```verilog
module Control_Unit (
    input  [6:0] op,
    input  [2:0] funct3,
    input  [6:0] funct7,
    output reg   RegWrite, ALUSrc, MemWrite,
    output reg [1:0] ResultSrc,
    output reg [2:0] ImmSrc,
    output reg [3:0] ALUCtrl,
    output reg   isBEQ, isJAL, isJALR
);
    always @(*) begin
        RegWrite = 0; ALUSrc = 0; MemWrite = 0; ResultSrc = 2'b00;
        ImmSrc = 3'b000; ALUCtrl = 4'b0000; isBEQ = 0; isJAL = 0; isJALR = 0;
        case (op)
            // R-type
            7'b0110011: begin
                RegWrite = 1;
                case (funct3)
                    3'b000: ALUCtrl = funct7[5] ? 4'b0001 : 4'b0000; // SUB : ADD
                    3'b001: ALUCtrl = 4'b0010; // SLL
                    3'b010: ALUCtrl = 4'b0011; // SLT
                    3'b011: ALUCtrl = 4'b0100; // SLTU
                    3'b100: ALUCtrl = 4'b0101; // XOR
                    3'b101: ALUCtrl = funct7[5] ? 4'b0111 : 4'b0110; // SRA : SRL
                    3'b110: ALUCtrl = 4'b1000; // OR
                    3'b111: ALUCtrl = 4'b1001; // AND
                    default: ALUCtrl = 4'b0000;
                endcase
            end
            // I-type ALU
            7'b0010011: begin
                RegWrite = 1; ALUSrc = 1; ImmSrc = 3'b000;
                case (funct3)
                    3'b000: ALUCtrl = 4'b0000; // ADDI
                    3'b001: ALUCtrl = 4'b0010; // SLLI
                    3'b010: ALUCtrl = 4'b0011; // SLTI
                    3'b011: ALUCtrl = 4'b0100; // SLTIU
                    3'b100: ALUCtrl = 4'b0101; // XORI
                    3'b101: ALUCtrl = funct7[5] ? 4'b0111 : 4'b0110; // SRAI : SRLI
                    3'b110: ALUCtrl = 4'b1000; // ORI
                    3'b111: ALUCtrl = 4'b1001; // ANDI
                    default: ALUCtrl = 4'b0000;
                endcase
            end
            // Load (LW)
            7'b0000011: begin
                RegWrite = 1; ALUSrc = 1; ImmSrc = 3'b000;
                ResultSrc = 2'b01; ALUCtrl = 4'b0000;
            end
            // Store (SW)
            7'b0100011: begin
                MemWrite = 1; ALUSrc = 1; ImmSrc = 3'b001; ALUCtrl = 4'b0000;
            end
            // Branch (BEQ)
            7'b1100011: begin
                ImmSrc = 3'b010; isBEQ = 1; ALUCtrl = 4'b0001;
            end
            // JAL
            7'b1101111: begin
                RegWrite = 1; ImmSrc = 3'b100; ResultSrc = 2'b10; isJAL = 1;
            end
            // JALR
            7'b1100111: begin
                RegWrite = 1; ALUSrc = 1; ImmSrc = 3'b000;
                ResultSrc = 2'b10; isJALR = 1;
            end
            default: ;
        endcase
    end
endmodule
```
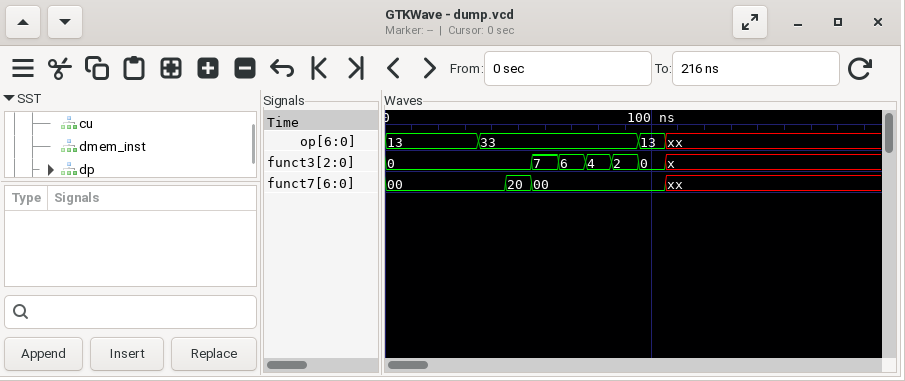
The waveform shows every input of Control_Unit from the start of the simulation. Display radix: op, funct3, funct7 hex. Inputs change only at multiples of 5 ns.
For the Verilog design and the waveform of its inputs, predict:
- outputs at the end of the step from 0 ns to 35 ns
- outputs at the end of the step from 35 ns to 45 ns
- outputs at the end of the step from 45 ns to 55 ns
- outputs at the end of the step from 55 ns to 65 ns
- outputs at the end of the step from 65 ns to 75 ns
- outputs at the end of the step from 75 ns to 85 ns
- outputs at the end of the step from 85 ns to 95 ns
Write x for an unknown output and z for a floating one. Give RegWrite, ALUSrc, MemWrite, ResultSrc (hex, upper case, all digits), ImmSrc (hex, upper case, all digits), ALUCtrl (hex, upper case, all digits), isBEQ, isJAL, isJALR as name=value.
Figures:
RegWrite=1, ALUSrc=1, MemWrite=0, ResultSrc=0, ImmSrc=0, ALUCtrl=0, isBEQ=0, isJAL=0, isJALR=0
RegWrite=1, ALUSrc=0, MemWrite=0, ResultSrc=0, ImmSrc=0, ALUCtrl=0, isBEQ=0, isJAL=0, isJALR=0
RegWrite=1, ALUSrc=0, MemWrite=0, ResultSrc=0, ImmSrc=0, ALUCtrl=1, isBEQ=0, isJAL=0, isJALR=0
RegWrite=1, ALUSrc=0, MemWrite=0, ResultSrc=0, ImmSrc=0, ALUCtrl=9, isBEQ=0, isJAL=0, isJALR=0
RegWrite=1, ALUSrc=0, MemWrite=0, ResultSrc=0, ImmSrc=0, ALUCtrl=8, isBEQ=0, isJAL=0, isJALR=0
RegWrite=1, ALUSrc=0, MemWrite=0, ResultSrc=0, ImmSrc=0, ALUCtrl=5, isBEQ=0, isJAL=0, isJALR=0
RegWrite=1, ALUSrc=0, MemWrite=0, ResultSrc=0, ImmSrc=0, ALUCtrl=3, isBEQ=0, isJAL=0, isJALR=0
